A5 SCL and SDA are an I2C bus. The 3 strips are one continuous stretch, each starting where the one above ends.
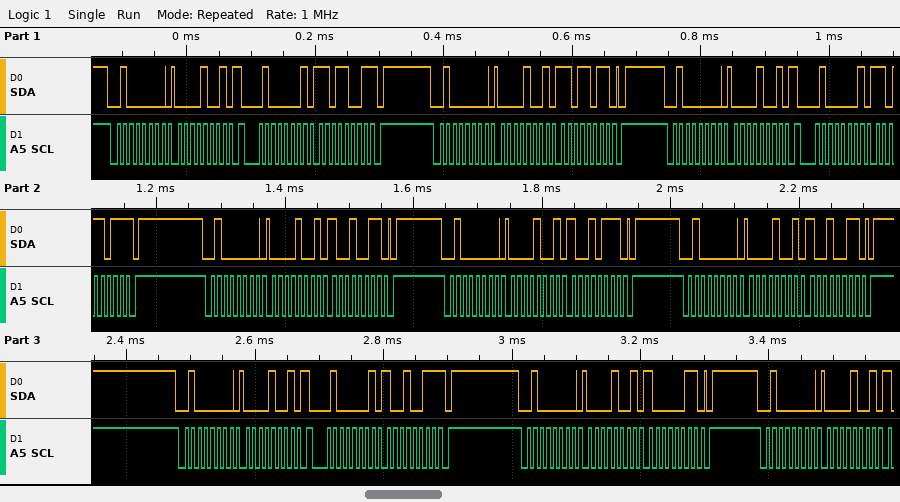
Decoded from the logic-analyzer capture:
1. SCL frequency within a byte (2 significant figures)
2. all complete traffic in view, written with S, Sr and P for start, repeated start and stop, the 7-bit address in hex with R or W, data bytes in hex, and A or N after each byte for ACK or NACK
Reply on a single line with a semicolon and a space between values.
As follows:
100 kHz; S 20W A 09 A Sr 20R A D9 N P S 20W A 09 A DB A P S 20W A 09 A Sr 20R A DB N P S 20W A 09 A 93 A P S 20W A 09 A 97 A P S 20W A 09 A 93 A P S 20W A 09 A Sr 20R A 93 N P S 20W A 09 A 83 A P S 20W A 09 A
